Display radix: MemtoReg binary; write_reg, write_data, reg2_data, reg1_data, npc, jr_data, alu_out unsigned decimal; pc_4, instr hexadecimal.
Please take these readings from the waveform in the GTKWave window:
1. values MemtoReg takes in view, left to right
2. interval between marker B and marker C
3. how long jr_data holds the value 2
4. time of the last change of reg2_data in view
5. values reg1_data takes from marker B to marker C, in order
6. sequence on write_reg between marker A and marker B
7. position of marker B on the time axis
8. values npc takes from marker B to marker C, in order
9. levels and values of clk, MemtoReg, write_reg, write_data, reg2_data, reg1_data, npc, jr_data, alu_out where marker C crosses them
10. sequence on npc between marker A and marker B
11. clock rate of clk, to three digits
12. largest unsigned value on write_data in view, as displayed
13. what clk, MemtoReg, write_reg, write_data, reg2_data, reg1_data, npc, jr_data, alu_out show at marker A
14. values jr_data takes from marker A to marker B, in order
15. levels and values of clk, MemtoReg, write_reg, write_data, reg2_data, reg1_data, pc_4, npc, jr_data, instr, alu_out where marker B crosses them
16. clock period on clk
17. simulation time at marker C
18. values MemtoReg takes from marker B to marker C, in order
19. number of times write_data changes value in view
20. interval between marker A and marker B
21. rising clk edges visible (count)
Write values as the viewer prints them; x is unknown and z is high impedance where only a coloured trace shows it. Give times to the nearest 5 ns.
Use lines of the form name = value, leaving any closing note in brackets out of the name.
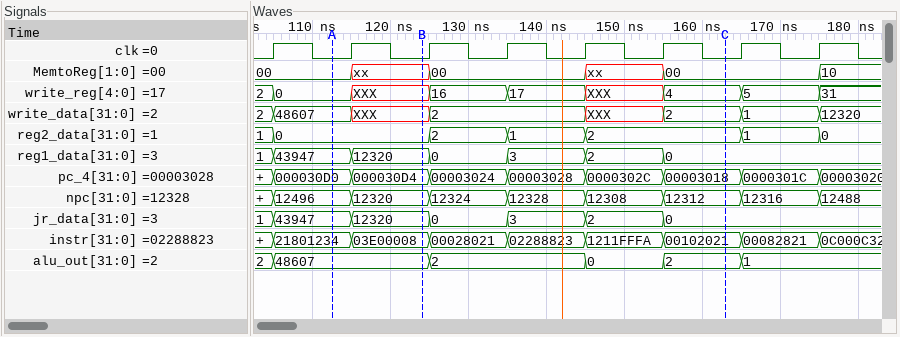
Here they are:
values MemtoReg takes in view, left to right = 00, xx, 00, xx, 00, 10
interval between marker B and marker C = 40 ns
how long jr_data holds the value 2 = 10 ns
time of the last change of reg2_data in view = 175 ns
values reg1_data takes from marker B to marker C, in order = 12320, 0, 3, 2, 0
sequence on write_reg between marker A and marker B = 0, XXX
position of marker B on the time axis = 125 ns
values npc takes from marker B to marker C, in order = 12320, 12324, 12328, 12308, 12312
levels and values of clk, MemtoReg, write_reg, write_data, reg2_data, reg1_data, npc, jr_data, alu_out where marker C crosses them = clk=0, MemtoReg=00, write_reg=4, write_data=2, reg2_data=2, reg1_data=0, npc=12312, jr_data=0, alu_out=2
sequence on npc between marker A and marker B = 12496, 12320
clock rate of clk, to three digits = 100 MHz
largest unsigned value on write_data in view, as displayed = 48607
what clk, MemtoReg, write_reg, write_data, reg2_data, reg1_data, npc, jr_data, alu_out show at marker A = clk=0, MemtoReg=00, write_reg=0, write_data=48607, reg2_data=0, reg1_data=43947, npc=12496, jr_data=43947, alu_out=48607
values jr_data takes from marker A to marker B, in order = 43947, 12320
levels and values of clk, MemtoReg, write_reg, write_data, reg2_data, reg1_data, pc_4, npc, jr_data, instr, alu_out where marker B crosses them = clk=0, MemtoReg=xx, write_reg=XXX, write_data=XXX, reg2_data=0, reg1_data=12320, pc_4=000030D4, npc=12320, jr_data=12320, instr=03E00008, alu_out=48607
clock period on clk = 10 ns
simulation time at marker C = 165 ns
values MemtoReg takes from marker B to marker C, in order = xx, 00, xx, 00
number of times write_data changes value in view = 7
interval between marker A and marker B = 10 ns
rising clk edges visible = 8
